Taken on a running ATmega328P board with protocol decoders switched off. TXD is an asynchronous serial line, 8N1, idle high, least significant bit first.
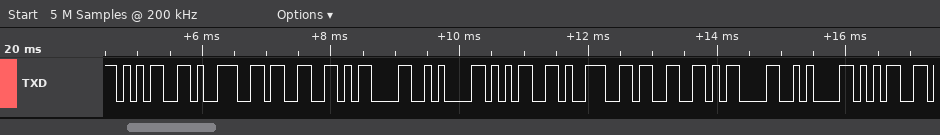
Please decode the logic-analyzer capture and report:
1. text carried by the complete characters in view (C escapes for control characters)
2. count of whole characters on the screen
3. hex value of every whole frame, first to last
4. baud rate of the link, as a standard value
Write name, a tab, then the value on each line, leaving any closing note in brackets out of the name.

text carried by the complete characters in view	"593\r\n593\r\n5"
count of whole characters on the screen	11
hex value of every whole frame, first to last	0x35 0x39 0x33 0x0D 0x0A 0x35 0x39 0x33 0x0D 0x0A 0x35
baud rate of the link, as a standard value	9600 baud
